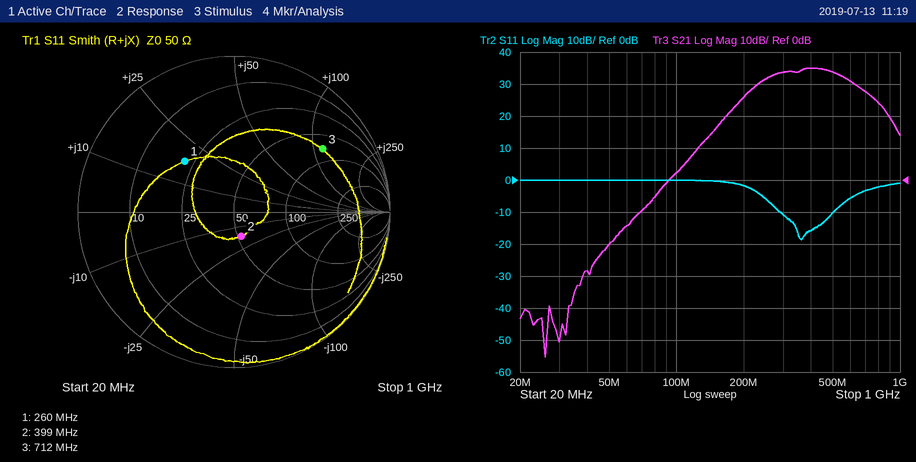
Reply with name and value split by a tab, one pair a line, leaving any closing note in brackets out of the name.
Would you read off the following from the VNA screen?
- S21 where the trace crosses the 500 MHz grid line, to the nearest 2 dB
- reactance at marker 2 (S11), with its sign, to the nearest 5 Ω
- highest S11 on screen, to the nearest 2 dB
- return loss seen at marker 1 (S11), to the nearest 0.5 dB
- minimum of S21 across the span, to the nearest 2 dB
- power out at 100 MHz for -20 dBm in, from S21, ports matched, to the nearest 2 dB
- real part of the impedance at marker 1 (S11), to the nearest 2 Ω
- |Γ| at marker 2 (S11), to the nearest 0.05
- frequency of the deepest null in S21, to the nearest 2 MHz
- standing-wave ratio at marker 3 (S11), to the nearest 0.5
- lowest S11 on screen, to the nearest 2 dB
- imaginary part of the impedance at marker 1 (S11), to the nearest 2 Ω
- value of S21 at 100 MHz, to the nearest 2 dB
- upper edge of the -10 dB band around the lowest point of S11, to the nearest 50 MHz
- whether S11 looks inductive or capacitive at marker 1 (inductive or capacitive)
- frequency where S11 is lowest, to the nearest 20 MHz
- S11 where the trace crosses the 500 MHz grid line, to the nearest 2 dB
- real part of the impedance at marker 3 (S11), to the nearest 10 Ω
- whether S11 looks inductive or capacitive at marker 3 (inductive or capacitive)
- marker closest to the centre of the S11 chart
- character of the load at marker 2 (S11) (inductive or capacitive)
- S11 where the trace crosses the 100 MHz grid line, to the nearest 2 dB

S21 where the trace crosses the 500 MHz grid line, to the nearest 2 dB	34 dB
reactance at marker 2 (S11), with its sign, to the nearest 5 Ω	-15 Ω
highest S11 on screen, to the nearest 2 dB	0 dB
return loss seen at marker 1 (S11), to the nearest 0.5 dB	7.0 dB
minimum of S21 across the span, to the nearest 2 dB	-56 dB
power out at 100 MHz for -20 dBm in, from S21, ports matched, to the nearest 2 dB	-18 dBm
real part of the impedance at marker 1 (S11), to the nearest 2 Ω	22 Ω
|Γ| at marker 2 (S11), to the nearest 0.05	0.15
frequency of the deepest null in S21, to the nearest 2 MHz	26 MHz
standing-wave ratio at marker 3 (S11), to the nearest 0.5	5.5
lowest S11 on screen, to the nearest 2 dB	-18 dB
imaginary part of the impedance at marker 1 (S11), to the nearest 2 Ω	+18 Ω
value of S21 at 100 MHz, to the nearest 2 dB	2 dB
upper edge of the -10 dB band around the lowest point of S11, to the nearest 50 MHz	500 MHz
whether S11 looks inductive or capacitive at marker 1	inductive
frequency where S11 is lowest, to the nearest 20 MHz	360 MHz
S11 where the trace crosses the 500 MHz grid line, to the nearest 2 dB	-10 dB
real part of the impedance at marker 3 (S11), to the nearest 10 Ω	70 Ω
whether S11 looks inductive or capacitive at marker 3	inductive
marker closest to the centre of the S11 chart	marker 2
character of the load at marker 2 (S11)	capacitive
S11 where the trace crosses the 100 MHz grid line, to the nearest 2 dB	0 dB
